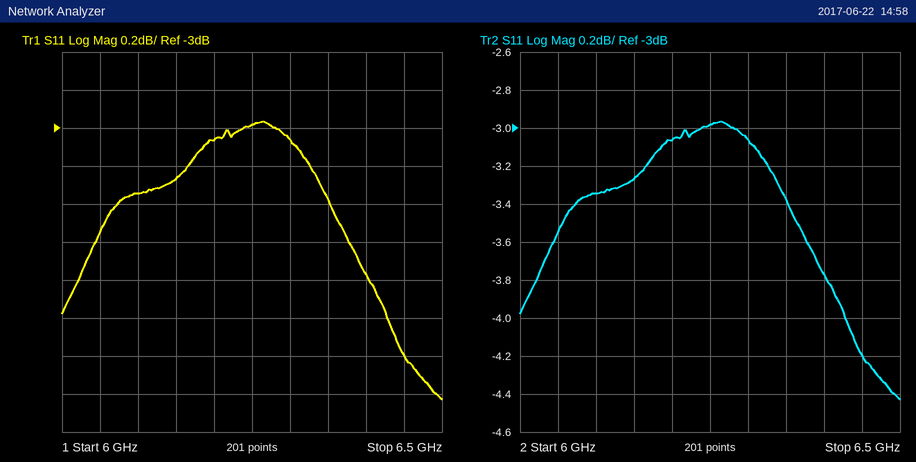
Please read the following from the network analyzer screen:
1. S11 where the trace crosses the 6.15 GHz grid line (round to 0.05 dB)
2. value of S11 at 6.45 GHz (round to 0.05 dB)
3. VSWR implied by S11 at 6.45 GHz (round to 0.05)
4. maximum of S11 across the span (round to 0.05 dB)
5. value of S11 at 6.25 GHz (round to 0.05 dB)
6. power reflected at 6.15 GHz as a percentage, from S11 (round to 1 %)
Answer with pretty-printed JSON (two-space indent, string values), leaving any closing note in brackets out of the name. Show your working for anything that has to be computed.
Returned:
{
  "S11 where the trace crosses the 6.15 GHz grid line": "-3.25 dB",
  "value of S11 at 6.45 GHz": "-4.20 dB",
  "VSWR implied by S11 at 6.45 GHz": "|Γ| = 10^(-4.2/20) = 0.6166; VSWR = (1 + 0.6166)/(1 − 0.6166) ≈ 4.22, so 4.20 to the nearest 0.05",
  "maximum of S11 across the span": "-2.95 dB",
  "value of S11 at 6.25 GHz": "-3.00 dB",
  "power reflected at 6.15 GHz as a percentage, from S11": "10^(-3.25/10) ≈ 47 %"
}
